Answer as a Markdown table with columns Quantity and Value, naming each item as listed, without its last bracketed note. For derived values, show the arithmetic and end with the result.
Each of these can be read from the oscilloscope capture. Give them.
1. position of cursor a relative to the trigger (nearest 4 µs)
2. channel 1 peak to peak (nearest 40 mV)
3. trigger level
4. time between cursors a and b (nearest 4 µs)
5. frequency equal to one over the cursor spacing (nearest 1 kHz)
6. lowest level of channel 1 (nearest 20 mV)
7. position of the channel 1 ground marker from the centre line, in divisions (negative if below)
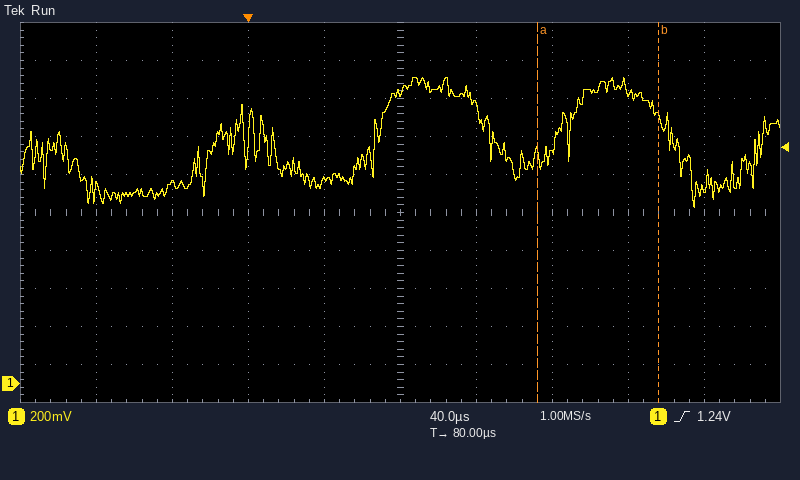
| Quantity | Value |
|---|---|
| position of cursor a relative to the trigger | +152 µs |
| channel 1 peak to peak | 680 mV |
| trigger level | 1.24 V |
| time between cursors a and b | 64 µs |
| frequency equal to one over the cursor spacing | 1 / 64 µs ≈ 16 kHz |
| lowest level of channel 1 | 920 mV |
| position of the channel 1 ground marker from the centre line, in divisions | -4.5 div |
